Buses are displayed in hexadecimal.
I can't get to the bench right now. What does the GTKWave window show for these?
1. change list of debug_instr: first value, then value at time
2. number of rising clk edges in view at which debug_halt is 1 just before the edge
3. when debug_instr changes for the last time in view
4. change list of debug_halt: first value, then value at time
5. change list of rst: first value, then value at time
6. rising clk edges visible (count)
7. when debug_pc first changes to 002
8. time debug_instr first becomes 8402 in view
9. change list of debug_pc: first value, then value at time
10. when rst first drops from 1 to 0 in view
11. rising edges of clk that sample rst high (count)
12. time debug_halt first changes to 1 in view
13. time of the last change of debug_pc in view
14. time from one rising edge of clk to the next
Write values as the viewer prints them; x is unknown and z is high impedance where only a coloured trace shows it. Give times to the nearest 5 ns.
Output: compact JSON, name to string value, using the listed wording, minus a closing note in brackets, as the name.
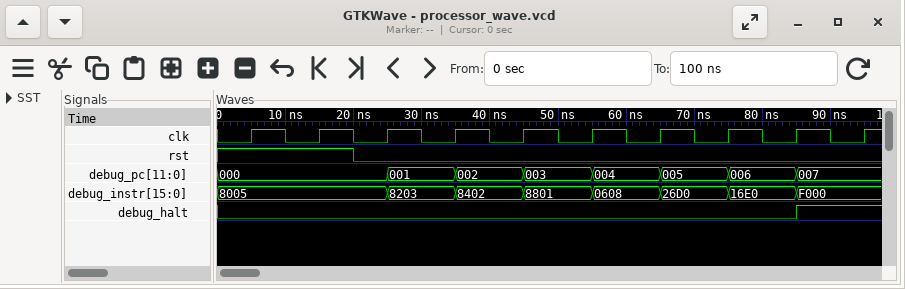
{"change list of debug_instr: first value, then value at time": "8005, 8203 at 25 ns, 8402 at 35 ns, 8801 at 45 ns, 0608 at 55 ns, 26D0 at 65 ns, 16E0 at 75 ns, F000 at 85 ns", "number of rising clk edges in view at which debug_halt is 1 just before the edge": "1", "when debug_instr changes for the last time in view": "85 ns", "change list of debug_halt: first value, then value at time": "0, 1 at 85 ns", "change list of rst: first value, then value at time": "1, 0 at 20 ns", "rising clk edges visible": "10", "when debug_pc first changes to 002": "35 ns", "time debug_instr first becomes 8402 in view": "35 ns", "change list of debug_pc: first value, then value at time": "000, 001 at 25 ns, 002 at 35 ns, 003 at 45 ns, 004 at 55 ns, 005 at 65 ns, 006 at 75 ns, 007 at 85 ns", "when rst first drops from 1 to 0 in view": "20 ns", "rising edges of clk that sample rst high": "2", "time debug_halt first changes to 1 in view": "85 ns", "time of the last change of debug_pc in view": "85 ns", "time from one rising edge of clk to the next": "10 ns"}
